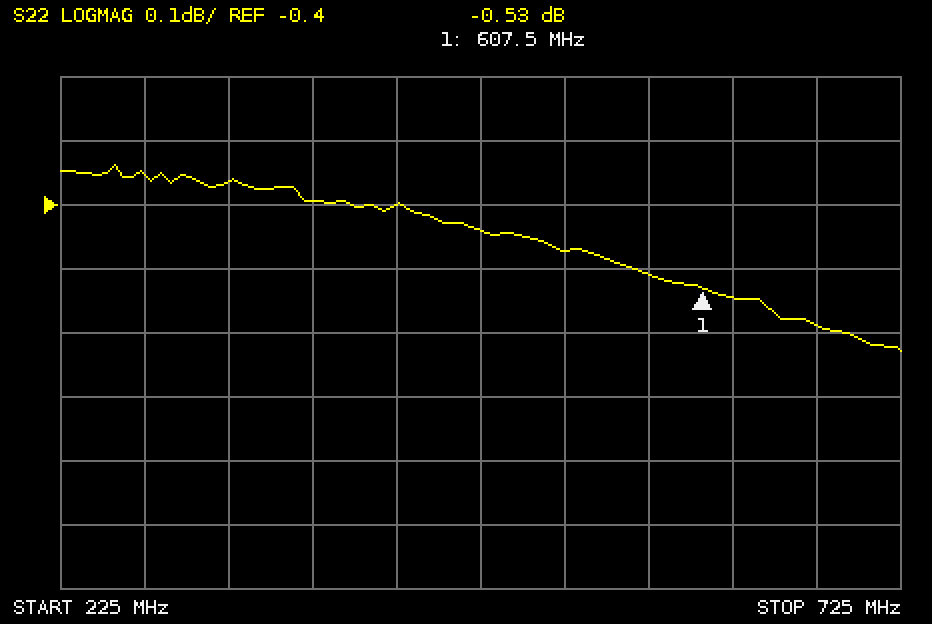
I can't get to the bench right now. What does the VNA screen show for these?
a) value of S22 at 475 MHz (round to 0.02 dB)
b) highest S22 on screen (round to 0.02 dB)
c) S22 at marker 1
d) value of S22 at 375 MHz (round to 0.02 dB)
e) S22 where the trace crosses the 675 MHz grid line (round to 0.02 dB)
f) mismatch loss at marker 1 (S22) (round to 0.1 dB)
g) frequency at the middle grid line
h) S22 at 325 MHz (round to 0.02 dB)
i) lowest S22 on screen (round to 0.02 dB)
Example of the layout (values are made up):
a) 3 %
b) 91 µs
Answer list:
a) -0.44 dB
b) -0.34 dB
c) -0.53 dB
d) -0.40 dB
e) -0.58 dB
f) 9.4 dB
g) 475 MHz
h) -0.36 dB
i) -0.62 dB
